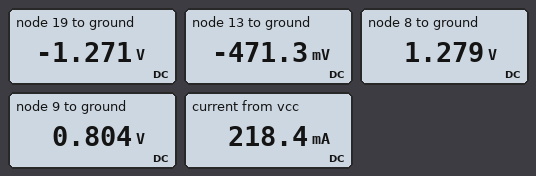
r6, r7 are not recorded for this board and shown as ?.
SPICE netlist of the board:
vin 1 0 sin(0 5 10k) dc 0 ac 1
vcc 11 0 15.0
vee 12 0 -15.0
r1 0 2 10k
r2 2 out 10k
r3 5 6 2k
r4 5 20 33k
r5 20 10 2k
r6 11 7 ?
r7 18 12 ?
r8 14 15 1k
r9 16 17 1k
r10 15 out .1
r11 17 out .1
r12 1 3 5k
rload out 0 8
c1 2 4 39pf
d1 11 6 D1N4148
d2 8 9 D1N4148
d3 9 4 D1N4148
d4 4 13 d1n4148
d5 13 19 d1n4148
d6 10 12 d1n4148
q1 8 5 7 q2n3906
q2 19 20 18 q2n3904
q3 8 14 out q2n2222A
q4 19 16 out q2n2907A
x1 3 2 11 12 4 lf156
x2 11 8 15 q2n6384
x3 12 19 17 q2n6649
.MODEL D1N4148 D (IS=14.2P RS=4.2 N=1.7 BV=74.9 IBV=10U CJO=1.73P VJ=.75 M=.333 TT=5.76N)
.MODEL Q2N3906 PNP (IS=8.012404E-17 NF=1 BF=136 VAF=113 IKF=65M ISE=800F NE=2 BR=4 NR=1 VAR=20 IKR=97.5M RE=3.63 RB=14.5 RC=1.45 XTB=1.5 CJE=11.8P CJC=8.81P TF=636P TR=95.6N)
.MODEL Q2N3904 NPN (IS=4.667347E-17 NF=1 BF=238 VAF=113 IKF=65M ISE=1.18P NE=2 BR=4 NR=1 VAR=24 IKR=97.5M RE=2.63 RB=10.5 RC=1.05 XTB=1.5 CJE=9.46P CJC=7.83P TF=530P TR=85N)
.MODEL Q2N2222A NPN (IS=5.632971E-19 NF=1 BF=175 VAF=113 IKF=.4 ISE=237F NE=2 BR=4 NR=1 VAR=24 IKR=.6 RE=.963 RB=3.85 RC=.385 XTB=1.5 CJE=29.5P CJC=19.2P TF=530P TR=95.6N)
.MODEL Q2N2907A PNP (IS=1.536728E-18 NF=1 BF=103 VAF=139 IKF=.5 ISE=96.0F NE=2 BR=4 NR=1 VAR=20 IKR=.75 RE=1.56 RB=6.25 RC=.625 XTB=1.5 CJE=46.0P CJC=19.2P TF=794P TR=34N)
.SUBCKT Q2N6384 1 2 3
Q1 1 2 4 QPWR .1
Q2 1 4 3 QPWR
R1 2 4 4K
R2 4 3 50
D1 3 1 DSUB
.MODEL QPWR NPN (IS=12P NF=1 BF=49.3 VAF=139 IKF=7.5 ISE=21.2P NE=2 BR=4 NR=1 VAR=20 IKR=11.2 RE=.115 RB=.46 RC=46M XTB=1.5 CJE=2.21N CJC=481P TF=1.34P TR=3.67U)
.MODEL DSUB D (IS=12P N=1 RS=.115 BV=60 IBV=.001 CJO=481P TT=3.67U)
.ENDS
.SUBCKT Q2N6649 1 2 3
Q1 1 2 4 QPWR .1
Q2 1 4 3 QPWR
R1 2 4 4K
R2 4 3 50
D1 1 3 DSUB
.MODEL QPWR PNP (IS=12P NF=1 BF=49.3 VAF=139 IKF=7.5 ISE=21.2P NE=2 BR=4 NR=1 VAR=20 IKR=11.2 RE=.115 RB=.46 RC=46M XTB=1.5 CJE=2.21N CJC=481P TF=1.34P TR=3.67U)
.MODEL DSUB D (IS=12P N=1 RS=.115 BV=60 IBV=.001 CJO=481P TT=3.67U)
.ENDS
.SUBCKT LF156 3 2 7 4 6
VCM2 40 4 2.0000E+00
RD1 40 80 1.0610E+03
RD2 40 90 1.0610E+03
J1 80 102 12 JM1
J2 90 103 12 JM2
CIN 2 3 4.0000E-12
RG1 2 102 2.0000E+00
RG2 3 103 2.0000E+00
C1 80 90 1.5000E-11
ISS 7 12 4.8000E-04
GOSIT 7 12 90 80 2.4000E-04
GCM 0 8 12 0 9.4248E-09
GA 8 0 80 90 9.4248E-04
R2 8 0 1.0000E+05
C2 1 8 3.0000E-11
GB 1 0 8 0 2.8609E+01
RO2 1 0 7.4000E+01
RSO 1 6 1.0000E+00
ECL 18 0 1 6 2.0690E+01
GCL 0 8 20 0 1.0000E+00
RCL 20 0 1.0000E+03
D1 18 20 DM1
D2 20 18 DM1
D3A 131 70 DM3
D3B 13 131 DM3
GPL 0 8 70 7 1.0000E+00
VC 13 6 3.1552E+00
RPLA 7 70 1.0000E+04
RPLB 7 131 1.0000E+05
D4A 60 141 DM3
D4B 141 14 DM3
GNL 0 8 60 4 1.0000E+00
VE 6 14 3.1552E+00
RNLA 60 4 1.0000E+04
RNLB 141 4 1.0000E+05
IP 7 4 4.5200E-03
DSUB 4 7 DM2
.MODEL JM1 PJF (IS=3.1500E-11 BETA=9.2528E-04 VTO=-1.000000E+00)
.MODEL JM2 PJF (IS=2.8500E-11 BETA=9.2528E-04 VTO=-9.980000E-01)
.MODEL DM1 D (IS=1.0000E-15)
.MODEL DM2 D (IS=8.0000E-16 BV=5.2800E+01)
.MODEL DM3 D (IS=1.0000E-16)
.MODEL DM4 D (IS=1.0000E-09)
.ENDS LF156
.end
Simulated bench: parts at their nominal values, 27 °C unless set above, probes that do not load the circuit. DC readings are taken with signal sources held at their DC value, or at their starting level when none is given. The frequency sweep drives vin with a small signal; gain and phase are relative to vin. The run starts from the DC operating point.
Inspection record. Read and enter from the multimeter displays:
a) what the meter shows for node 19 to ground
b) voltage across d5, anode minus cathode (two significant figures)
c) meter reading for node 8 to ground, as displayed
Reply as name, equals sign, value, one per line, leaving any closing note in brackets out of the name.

what the meter shows for node 19 to ground = -1.271 V
voltage across d5, anode minus cathode = 800 mV
meter reading for node 8 to ground, as displayed = 1.279 V
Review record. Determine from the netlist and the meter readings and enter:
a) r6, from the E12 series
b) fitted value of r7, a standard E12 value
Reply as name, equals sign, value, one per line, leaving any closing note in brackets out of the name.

r6, from the E12 series = 3.3 kΩ
fitted value of r7, a standard E12 value = 1 kΩ
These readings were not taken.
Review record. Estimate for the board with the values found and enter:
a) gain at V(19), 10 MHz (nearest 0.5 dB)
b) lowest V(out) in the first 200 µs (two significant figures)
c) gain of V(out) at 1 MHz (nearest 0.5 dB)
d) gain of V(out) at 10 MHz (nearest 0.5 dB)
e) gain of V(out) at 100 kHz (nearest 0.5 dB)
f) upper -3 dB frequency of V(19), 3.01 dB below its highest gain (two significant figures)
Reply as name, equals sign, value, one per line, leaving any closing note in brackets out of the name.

gain at V(19), 10 MHz = -17.0 dB
lowest V(out) in the first 200 µs = -10 V
gain of V(out) at 1 MHz = 1.0 dB
gain of V(out) at 10 MHz = -19.5 dB
gain of V(out) at 100 kHz = 6.0 dB
upper -3 dB frequency of V(19), 3.01 dB below its highest gain = 530 kHz
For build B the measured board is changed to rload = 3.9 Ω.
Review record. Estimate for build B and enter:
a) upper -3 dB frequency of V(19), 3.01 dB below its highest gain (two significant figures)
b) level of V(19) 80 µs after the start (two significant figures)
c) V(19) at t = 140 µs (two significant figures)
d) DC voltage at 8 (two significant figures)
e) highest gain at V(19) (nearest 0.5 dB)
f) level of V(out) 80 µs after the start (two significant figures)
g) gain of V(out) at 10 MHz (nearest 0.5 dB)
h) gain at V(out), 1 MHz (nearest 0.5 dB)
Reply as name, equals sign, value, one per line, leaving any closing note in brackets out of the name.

upper -3 dB frequency of V(19), 3.01 dB below its highest gain = 470 kHz
level of V(19) 80 µs after the start = -9.0 V
V(19) at t = 140 µs = 5.8 V
DC voltage at 8 = 1.3 V
highest gain at V(19) = 7.0 dB
level of V(out) 80 µs after the start = -7.2 V
gain of V(out) at 10 MHz = -20.0 dB
gain at V(out), 1 MHz = 0.5 dB
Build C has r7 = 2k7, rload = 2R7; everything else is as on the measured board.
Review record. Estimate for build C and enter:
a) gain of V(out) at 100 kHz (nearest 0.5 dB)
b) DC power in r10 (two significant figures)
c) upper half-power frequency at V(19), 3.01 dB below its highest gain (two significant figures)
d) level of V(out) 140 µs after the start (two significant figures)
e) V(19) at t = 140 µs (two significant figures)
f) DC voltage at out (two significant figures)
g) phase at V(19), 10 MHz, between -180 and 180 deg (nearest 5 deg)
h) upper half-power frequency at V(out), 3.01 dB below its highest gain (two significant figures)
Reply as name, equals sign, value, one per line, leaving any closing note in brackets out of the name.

gain of V(out) at 100 kHz = 5.5 dB
DC power in r10 = 4.0 mW
upper half-power frequency at V(19), 3.01 dB below its highest gain = 400 kHz
level of V(out) 140 µs after the start = 630 mV
V(19) at t = 140 µs = 5.7 V
DC voltage at out = 4.0 mV
phase at V(19), 10 MHz, between -180 and 180 deg = 100 deg
upper half-power frequency at V(out), 3.01 dB below its highest gain = 390 kHz
